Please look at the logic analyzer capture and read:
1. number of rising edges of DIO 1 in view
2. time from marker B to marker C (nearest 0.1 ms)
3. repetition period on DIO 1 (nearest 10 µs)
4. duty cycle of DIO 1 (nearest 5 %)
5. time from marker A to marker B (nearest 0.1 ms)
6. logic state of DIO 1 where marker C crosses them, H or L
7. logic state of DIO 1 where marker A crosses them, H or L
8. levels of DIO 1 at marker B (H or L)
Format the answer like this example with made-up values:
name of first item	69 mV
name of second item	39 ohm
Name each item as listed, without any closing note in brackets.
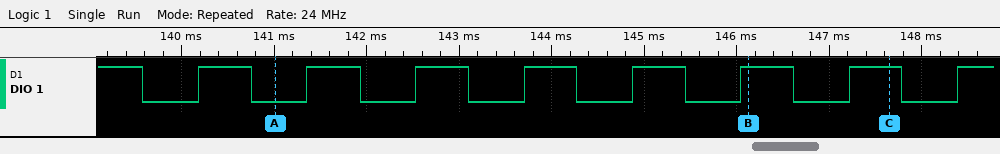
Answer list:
number of rising edges of DIO 1 in view	8
time from marker B to marker C	1.5 ms
repetition period on DIO 1	1170 µs
duty cycle of DIO 1	50 %
time from marker A to marker B	5.1 ms
logic state of DIO 1 where marker C crosses them, H or L	DIO 1=H
logic state of DIO 1 where marker A crosses them, H or L	DIO 1=L
levels of DIO 1 at marker B	DIO 1=H
